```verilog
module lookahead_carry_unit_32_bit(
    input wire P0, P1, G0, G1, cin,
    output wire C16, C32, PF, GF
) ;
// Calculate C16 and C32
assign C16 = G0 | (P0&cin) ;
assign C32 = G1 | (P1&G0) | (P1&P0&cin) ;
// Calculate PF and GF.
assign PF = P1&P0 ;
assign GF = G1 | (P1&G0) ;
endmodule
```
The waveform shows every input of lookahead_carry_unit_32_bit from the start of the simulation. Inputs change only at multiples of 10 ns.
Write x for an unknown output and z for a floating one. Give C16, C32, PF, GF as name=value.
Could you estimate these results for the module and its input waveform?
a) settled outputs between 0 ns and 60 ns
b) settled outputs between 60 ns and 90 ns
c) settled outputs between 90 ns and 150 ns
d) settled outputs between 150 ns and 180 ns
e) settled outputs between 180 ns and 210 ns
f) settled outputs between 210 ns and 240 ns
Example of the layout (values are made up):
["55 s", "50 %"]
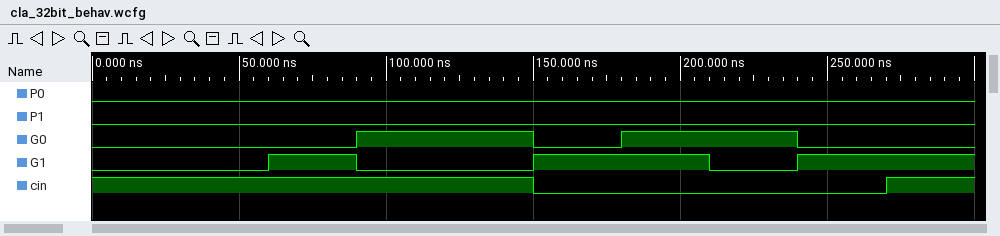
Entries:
["C16=0, C32=0, PF=0, GF=0", "C16=0, C32=1, PF=0, GF=1", "C16=1, C32=0, PF=0, GF=0", "C16=0, C32=1, PF=0, GF=1", "C16=1, C32=1, PF=0, GF=1", "C16=1, C32=0, PF=0, GF=0"]
